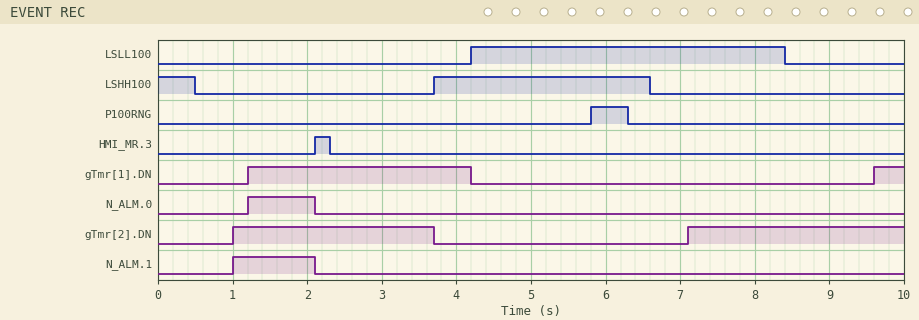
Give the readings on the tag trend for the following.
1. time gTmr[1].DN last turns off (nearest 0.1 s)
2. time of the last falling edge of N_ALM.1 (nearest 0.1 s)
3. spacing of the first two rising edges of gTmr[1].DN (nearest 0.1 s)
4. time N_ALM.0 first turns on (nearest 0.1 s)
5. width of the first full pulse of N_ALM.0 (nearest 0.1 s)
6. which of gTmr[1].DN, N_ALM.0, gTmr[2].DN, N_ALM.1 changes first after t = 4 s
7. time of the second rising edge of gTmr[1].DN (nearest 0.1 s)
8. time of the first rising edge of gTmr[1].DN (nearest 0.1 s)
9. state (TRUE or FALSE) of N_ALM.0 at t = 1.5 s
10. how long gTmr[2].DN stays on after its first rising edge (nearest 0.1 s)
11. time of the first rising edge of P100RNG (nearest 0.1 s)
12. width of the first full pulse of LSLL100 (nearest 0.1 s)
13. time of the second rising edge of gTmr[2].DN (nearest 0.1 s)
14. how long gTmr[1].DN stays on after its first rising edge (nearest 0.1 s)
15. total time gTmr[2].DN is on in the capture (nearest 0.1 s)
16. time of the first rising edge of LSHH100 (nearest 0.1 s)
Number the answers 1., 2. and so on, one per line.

1. 4.2 s
2. 2.1 s
3. 8.4 s
4. 1.2 s
5. 0.9 s
6. gTmr[1].DN
7. 9.6 s
8. 1.2 s
9. TRUE
10. 2.7 s
11. 5.8 s
12. 4.2 s
13. 7.1 s
14. 3.0 s
15. 5.6 s
16. 3.7 s
